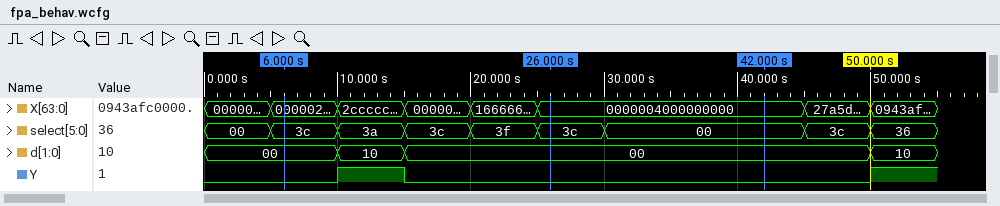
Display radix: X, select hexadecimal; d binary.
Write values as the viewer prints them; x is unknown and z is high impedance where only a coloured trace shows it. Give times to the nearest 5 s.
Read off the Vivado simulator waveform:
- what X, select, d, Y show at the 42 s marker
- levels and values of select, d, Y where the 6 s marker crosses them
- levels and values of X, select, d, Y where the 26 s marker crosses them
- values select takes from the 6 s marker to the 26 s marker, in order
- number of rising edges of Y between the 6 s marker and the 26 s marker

X=0000004000000000, select=00, d=00, Y=0
select=3c, d=00, Y=0
X=0000004000000000, select=3c, d=00, Y=0
3c, 3a, 3c, 3f, 3c
1
